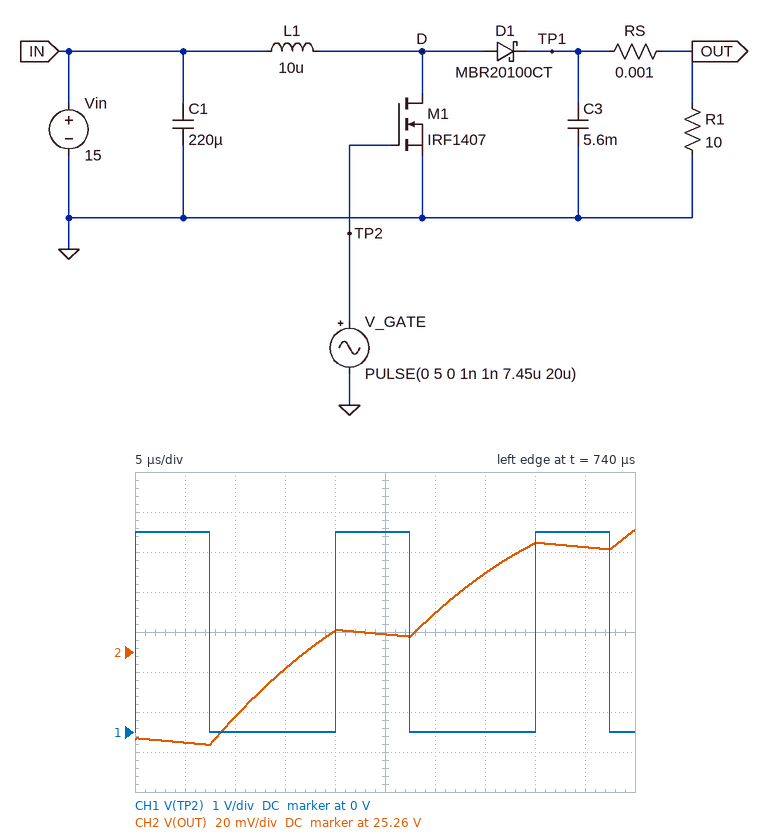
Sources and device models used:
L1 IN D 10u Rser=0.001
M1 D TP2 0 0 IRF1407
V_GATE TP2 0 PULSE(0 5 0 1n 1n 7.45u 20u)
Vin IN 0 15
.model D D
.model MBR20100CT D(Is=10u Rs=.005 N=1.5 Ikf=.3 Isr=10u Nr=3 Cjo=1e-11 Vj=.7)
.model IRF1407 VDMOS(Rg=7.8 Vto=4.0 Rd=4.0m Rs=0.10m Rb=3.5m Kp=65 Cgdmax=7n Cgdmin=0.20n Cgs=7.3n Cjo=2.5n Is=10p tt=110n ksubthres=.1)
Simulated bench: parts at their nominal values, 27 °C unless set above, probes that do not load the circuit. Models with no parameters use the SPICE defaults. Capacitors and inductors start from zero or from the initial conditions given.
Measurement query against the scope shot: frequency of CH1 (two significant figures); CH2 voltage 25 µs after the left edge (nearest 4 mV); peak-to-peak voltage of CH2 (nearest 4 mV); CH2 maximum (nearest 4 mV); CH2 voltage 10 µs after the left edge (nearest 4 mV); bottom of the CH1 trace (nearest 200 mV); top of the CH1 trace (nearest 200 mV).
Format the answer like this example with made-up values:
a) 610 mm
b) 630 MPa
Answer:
a) 50 kHz
b) 25.268 V
c) 108 mV
d) 25.320 V
e) 25.228 V
f) 0 V
g) 5.0 V
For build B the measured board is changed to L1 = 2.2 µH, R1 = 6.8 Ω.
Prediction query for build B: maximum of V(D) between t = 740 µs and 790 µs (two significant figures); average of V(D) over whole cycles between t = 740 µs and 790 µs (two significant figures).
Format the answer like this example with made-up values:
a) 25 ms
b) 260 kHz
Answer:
a) 24 V
b) 15 V
